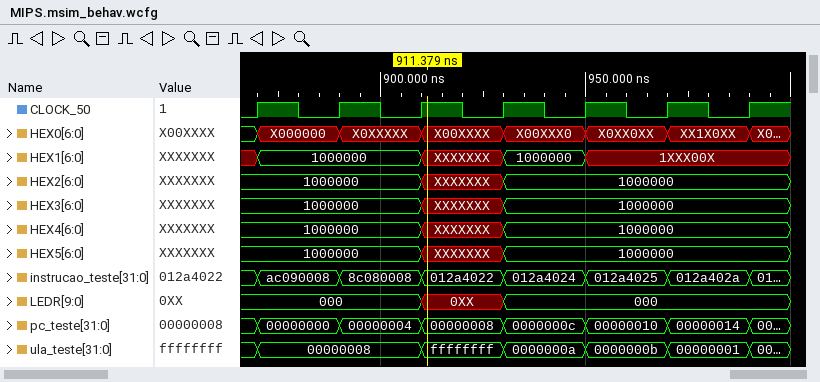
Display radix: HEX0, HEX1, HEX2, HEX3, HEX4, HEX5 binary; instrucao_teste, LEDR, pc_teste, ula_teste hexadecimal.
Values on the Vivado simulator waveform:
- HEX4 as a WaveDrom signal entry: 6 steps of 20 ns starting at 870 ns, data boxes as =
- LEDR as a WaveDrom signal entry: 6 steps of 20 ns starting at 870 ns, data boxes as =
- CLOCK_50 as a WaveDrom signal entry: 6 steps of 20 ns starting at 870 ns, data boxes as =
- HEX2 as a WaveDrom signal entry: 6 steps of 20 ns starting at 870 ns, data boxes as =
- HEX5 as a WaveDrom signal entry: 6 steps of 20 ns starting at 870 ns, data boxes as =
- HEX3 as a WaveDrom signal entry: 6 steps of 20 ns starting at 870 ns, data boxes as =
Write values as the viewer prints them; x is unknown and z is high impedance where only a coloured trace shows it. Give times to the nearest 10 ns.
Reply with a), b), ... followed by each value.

a) {name: 'HEX4', wave: '=.x=..', data: '1000000 1000000'}
b) {name: 'LEDR', wave: '=.==..', data: '000 0XX 000'}
c) {name: 'CLOCK_50', wave: 'p.....'}
d) {name: 'HEX2', wave: '=.x=..', data: '1000000 1000000'}
e) {name: 'HEX5', wave: '=.x=..', data: '1000000 1000000'}
f) {name: 'HEX3', wave: '=.x=..', data: '1000000 1000000'}
